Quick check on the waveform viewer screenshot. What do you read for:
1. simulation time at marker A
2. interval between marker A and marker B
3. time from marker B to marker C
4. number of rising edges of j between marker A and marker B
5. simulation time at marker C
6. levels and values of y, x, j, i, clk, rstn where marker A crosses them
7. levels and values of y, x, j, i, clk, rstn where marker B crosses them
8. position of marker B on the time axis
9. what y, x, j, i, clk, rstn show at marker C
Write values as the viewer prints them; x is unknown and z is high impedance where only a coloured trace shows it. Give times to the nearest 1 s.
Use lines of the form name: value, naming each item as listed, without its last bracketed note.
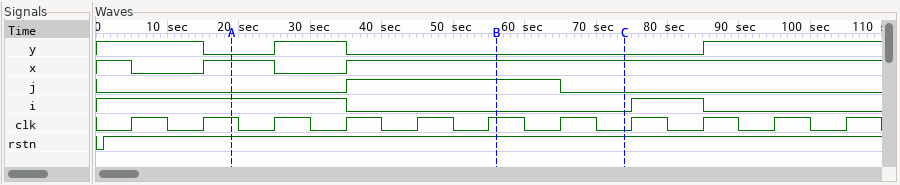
simulation time at marker A: 19 s
interval between marker A and marker B: 37 s
time from marker B to marker C: 18 s
number of rising edges of j between marker A and marker B: 1
simulation time at marker C: 74 s
levels and values of y, x, j, i, clk, rstn where marker A crosses them: y=0, x=1, j=0, i=1, clk=1, rstn=1
levels and values of y, x, j, i, clk, rstn where marker B crosses them: y=0, x=1, j=1, i=0, clk=1, rstn=1
position of marker B on the time axis: 56 s
what y, x, j, i, clk, rstn show at marker C: y=0, x=1, j=0, i=0, clk=0, rstn=1
